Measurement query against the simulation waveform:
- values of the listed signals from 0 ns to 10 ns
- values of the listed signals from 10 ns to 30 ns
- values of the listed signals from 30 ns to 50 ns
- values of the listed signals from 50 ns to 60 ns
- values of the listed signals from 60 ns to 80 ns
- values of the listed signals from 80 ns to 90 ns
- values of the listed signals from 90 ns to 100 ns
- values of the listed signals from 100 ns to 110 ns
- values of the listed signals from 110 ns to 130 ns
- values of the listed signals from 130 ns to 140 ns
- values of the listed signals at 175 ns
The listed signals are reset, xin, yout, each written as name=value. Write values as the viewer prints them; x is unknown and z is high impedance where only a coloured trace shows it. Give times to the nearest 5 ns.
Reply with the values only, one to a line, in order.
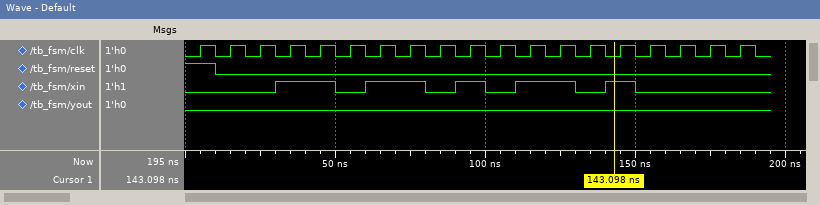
reset=1, xin=0, yout=0
reset=0, xin=0, yout=0
reset=0, xin=1, yout=0
reset=0, xin=0, yout=0
reset=0, xin=1, yout=0
reset=0, xin=0, yout=0
reset=0, xin=1, yout=0
reset=0, xin=0, yout=0
reset=0, xin=1, yout=0
reset=0, xin=0, yout=0
reset=0, xin=0, yout=0
